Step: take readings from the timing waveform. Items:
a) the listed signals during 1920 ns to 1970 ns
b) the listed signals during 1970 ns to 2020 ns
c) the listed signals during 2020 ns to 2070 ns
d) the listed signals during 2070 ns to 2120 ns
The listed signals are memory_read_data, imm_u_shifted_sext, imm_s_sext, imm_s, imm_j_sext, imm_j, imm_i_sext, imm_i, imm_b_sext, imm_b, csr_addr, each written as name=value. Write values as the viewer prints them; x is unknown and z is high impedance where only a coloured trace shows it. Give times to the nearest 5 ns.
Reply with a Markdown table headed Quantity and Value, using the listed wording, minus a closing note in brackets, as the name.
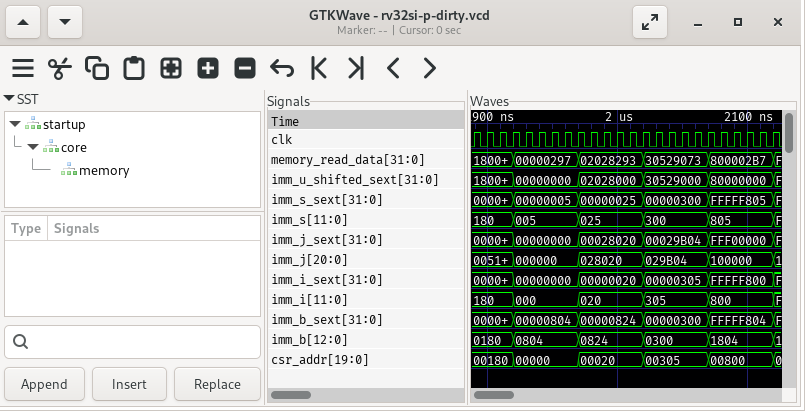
| Quantity | Value |
|---|---|
| the listed signals during 1920 ns to 1970 ns | memory_read_data=00000297, imm_u_shifted_sext=00000000, imm_s_sext=00000005, imm_s=005, imm_j_sext=00000000, imm_j=000000, imm_i_sext=00000000, imm_i=000, imm_b_sext=00000804, imm_b=0804, csr_addr=00000 |
| the listed signals during 1970 ns to 2020 ns | memory_read_data=02028293, imm_u_shifted_sext=02028000, imm_s_sext=00000025, imm_s=025, imm_j_sext=00028020, imm_j=028020, imm_i_sext=00000020, imm_i=020, imm_b_sext=00000824, imm_b=0824, csr_addr=00020 |
| the listed signals during 2020 ns to 2070 ns | memory_read_data=30529073, imm_u_shifted_sext=30529000, imm_s_sext=00000300, imm_s=300, imm_j_sext=00029B04, imm_j=029B04, imm_i_sext=00000305, imm_i=305, imm_b_sext=00000300, imm_b=0300, csr_addr=00305 |
| the listed signals during 2070 ns to 2120 ns | memory_read_data=800002B7, imm_u_shifted_sext=80000000, imm_s_sext=FFFFF805, imm_s=805, imm_j_sext=FFF00000, imm_j=100000, imm_i_sext=FFFFF800, imm_i=800, imm_b_sext=FFFFF804, imm_b=1804, csr_addr=00800 |
